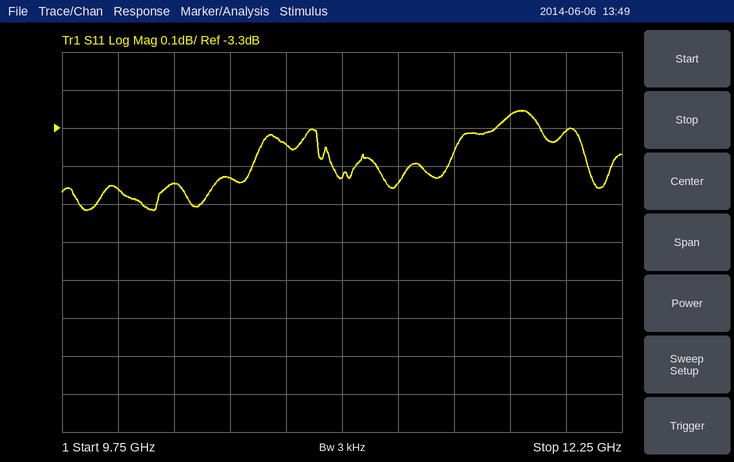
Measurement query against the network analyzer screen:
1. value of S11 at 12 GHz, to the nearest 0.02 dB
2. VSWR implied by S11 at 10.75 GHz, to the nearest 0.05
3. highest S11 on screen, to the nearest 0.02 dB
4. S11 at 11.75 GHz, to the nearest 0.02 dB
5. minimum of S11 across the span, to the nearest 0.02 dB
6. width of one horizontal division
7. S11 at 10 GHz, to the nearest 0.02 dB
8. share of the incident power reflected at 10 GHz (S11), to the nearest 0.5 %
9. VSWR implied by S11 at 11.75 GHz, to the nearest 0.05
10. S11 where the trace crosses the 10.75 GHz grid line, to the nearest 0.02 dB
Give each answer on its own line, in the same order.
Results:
-3.30 dB
5.25
-3.26 dB
-3.26 dB
-3.52 dB
250 MHz
-3.46 dB
45.0 %
5.40
-3.34 dB
